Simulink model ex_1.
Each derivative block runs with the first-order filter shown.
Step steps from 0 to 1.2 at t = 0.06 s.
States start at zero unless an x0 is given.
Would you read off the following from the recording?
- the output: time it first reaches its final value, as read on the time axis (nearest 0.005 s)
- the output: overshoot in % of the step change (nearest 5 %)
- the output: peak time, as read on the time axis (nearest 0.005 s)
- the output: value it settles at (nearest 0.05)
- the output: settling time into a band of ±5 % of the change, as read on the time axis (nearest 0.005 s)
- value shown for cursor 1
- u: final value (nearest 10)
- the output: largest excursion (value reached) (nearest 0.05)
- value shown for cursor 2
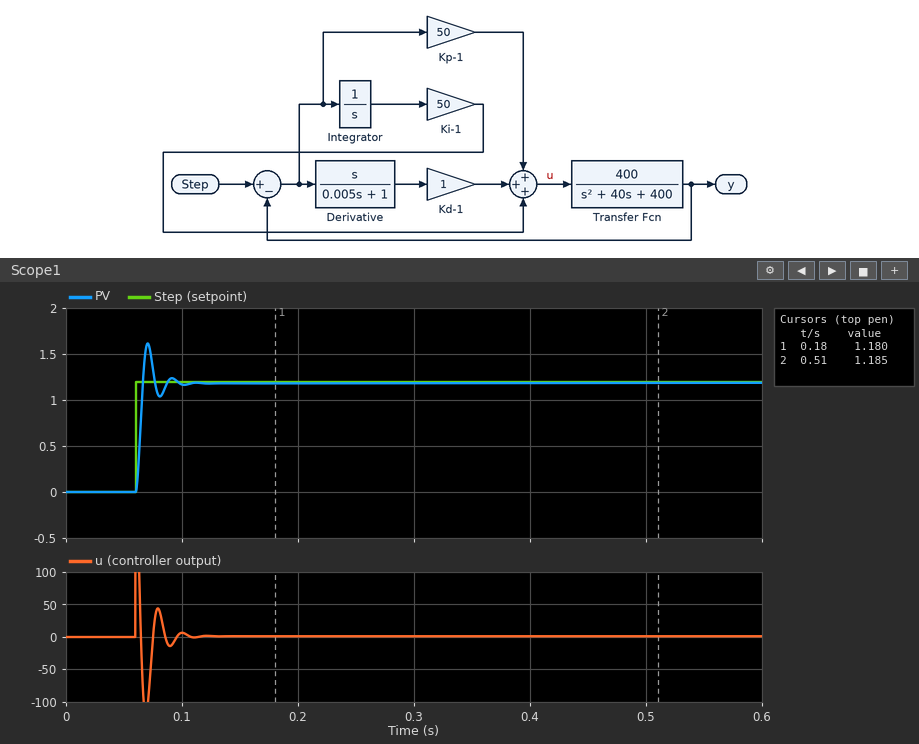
0.065 s
35 %
0.070 s
1.20
0.085 s
1.180
0
1.60
1.185
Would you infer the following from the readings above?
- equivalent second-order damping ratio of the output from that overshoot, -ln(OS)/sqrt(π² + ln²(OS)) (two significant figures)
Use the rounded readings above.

0.32
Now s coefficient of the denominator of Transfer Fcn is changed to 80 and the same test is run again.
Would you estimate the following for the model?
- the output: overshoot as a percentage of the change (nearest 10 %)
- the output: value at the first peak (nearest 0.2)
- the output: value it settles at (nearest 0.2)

20 %
1.4
1.2
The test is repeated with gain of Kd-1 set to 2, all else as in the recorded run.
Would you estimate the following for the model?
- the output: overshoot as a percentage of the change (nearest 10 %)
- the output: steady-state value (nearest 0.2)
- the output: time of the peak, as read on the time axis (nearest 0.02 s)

40 %
1.2
0.06 s
